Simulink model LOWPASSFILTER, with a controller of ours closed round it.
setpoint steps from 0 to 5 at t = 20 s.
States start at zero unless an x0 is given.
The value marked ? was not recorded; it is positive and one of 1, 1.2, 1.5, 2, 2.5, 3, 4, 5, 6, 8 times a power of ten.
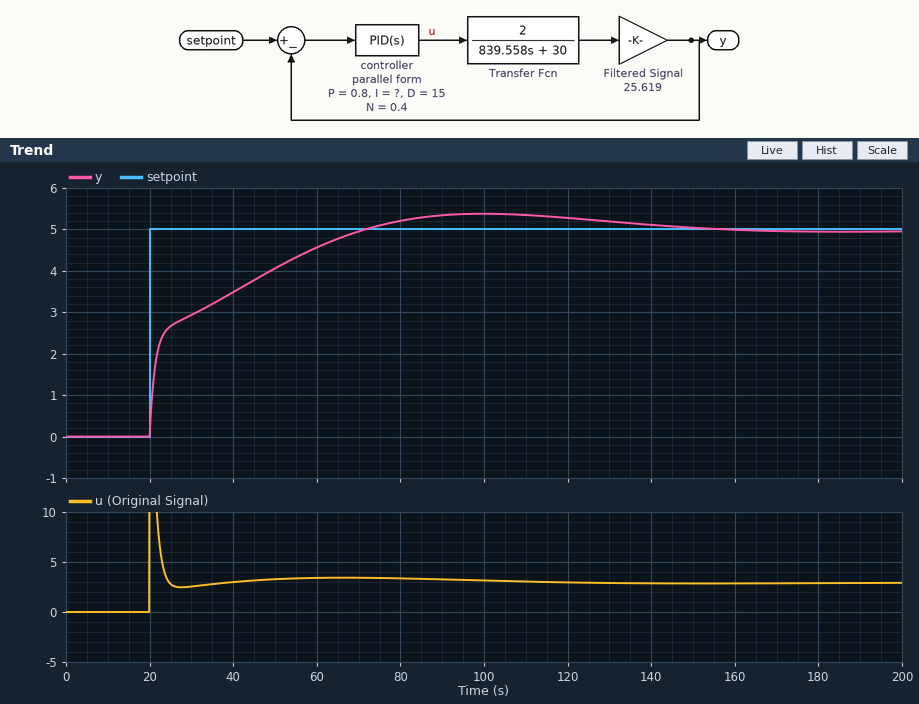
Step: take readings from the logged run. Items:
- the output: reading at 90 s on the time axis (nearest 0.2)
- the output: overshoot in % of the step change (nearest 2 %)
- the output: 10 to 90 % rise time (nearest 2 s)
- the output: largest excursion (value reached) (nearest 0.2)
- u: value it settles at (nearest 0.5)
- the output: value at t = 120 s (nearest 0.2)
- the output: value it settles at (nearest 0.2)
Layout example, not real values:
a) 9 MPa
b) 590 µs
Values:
a) 5.4
b) 8 %
c) 38 s
d) 5.4
e) 3.0
f) 5.2
g) 5.0
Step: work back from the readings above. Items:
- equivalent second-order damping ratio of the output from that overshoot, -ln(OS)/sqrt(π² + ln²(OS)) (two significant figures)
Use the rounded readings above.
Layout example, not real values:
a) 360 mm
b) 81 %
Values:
a) 0.63
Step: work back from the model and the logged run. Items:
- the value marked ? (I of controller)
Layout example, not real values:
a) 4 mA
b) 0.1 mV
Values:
a) 0.06
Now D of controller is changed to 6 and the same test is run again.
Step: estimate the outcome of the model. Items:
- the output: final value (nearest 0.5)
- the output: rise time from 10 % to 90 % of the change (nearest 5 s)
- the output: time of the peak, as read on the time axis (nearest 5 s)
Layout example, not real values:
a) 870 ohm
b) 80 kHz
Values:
a) 5.0
b) 30 s
c) 85 s
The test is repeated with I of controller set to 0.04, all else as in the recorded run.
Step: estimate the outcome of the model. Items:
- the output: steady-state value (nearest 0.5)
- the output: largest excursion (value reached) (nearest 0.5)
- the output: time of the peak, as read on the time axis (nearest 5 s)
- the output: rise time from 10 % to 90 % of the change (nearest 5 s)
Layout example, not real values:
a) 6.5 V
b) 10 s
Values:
a) 5.0
b) 5.0
c) 125 s
d) 50 s
